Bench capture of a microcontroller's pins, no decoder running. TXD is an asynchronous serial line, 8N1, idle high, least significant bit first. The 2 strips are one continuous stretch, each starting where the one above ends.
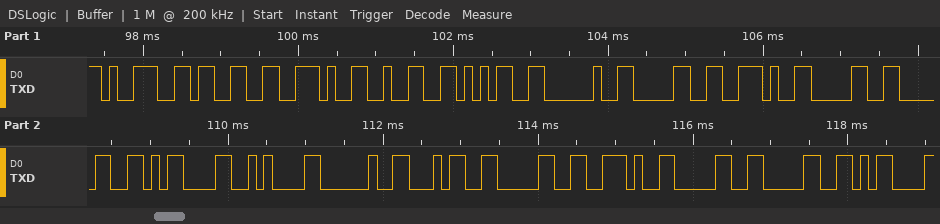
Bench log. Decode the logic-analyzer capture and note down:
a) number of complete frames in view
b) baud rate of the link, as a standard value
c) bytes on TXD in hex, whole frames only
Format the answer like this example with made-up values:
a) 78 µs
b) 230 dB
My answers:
a) 19
b) 9600 baud
c) 0x39 0x33 0x2E 0x32 0x35 0x20 0x30 0x2E 0x30 0x30 0x0D 0x0A 0x20 0x34 0x30 0x2E 0x30 0x30 0x0D
